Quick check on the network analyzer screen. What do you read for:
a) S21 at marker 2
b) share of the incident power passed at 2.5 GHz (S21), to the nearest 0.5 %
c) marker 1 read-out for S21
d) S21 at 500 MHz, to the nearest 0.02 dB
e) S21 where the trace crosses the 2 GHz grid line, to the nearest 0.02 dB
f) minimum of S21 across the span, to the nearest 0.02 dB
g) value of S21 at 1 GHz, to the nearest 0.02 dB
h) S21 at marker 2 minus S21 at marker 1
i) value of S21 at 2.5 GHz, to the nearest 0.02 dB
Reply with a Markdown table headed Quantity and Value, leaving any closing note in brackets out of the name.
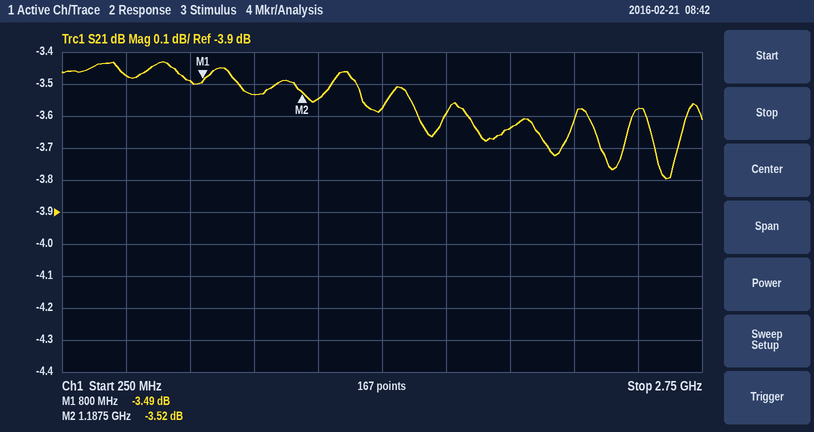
| Quantity | Value |
|---|---|
| S21 at marker 2 | -3.52 dB |
| share of the incident power passed at 2.5 GHz (S21), to the nearest 0.5 % | 44.0 % |
| marker 1 read-out for S21 | -3.49 dB |
| S21 at 500 MHz, to the nearest 0.02 dB | -3.48 dB |
| S21 where the trace crosses the 2 GHz grid line, to the nearest 0.02 dB | -3.64 dB |
| minimum of S21 across the span, to the nearest 0.02 dB | -3.80 dB |
| value of S21 at 1 GHz, to the nearest 0.02 dB | -3.54 dB |
| S21 at marker 2 minus S21 at marker 1 | -0.03 dB |
| value of S21 at 2.5 GHz, to the nearest 0.02 dB | -3.58 dB |
